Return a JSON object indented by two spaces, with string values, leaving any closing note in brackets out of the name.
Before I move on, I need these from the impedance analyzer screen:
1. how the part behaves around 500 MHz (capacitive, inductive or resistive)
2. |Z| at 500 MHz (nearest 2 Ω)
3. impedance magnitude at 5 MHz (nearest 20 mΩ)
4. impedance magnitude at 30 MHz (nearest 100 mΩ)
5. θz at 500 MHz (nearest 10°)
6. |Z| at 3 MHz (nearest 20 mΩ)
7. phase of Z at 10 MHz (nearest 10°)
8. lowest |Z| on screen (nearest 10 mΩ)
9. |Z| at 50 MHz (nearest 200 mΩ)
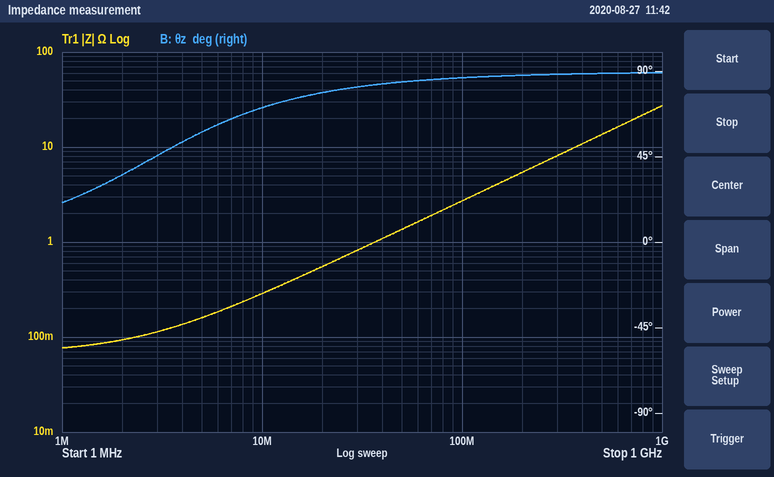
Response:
{
  "how the part behaves around 500 MHz": "inductive",
  "|Z| at 500 MHz": "14 Ω",
  "impedance magnitude at 5 MHz": "160 mΩ",
  "impedance magnitude at 30 MHz": "800 mΩ",
  "θz at 500 MHz": "90°",
  "|Z| at 3 MHz": "120 mΩ",
  "phase of Z at 10 MHz": "70°",
  "lowest |Z| on screen": "80 mΩ",
  "|Z| at 50 MHz": "1.4 Ω"
}
